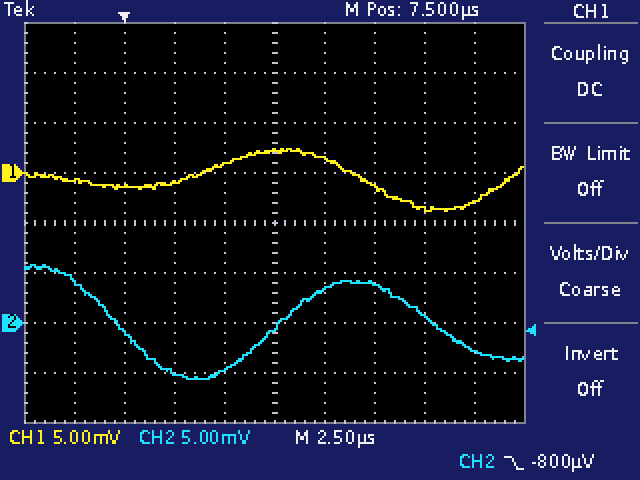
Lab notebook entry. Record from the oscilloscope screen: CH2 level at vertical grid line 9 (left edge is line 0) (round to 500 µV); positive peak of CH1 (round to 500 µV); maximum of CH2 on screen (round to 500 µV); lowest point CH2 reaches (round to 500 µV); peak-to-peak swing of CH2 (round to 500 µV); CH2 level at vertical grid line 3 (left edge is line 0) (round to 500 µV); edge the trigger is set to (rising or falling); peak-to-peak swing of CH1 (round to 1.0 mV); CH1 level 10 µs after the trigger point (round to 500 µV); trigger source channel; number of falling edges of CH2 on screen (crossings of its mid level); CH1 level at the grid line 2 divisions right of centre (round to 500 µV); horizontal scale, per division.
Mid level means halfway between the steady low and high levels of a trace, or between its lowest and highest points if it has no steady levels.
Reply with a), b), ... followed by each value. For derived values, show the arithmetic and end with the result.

a) -3.0 mV
b) 2.5 mV
c) 6.0 mV
d) -5.5 mV
e) 6.0 mV − (-5.5 mV) = 11.5 mV
f) -5.0 mV
g) falling
h) 6.0 mV
i) 1.5 mV
j) CH2
k) 2
l) -1.5 mV
m) 2.5 µs
